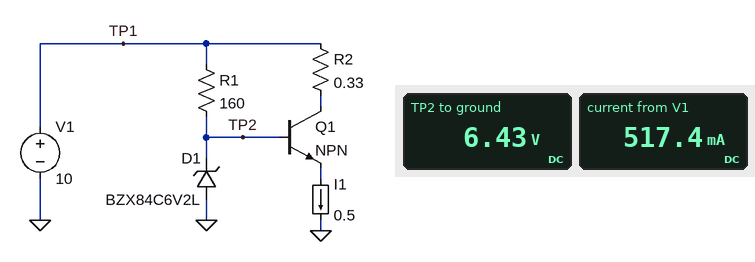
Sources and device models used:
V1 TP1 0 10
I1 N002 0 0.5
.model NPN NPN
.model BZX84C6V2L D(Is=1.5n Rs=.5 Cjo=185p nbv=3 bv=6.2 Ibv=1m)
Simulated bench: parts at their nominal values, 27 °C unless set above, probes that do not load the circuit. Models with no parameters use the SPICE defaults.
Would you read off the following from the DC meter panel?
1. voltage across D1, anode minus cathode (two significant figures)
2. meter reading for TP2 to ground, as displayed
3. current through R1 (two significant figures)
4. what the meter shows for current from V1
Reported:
-6.4 V
6.43 V
22 mA
517.4 mA
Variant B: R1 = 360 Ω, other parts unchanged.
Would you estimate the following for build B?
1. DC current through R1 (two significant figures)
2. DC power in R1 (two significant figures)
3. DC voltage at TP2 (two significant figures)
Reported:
10 mA
37 mW
6.3 V
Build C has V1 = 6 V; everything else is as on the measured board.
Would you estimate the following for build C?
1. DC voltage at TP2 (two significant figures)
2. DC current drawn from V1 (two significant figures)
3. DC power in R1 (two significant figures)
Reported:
5.2 V
500 mA
3.9 mW
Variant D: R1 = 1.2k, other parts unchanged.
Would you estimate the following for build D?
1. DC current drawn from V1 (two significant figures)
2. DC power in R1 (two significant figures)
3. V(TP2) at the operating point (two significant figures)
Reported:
500 mA
29 mW
4.1 V
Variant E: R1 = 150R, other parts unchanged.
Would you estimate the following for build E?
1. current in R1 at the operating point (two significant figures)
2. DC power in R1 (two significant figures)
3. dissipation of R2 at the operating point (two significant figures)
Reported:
24 mA
85 mW
81 mW
